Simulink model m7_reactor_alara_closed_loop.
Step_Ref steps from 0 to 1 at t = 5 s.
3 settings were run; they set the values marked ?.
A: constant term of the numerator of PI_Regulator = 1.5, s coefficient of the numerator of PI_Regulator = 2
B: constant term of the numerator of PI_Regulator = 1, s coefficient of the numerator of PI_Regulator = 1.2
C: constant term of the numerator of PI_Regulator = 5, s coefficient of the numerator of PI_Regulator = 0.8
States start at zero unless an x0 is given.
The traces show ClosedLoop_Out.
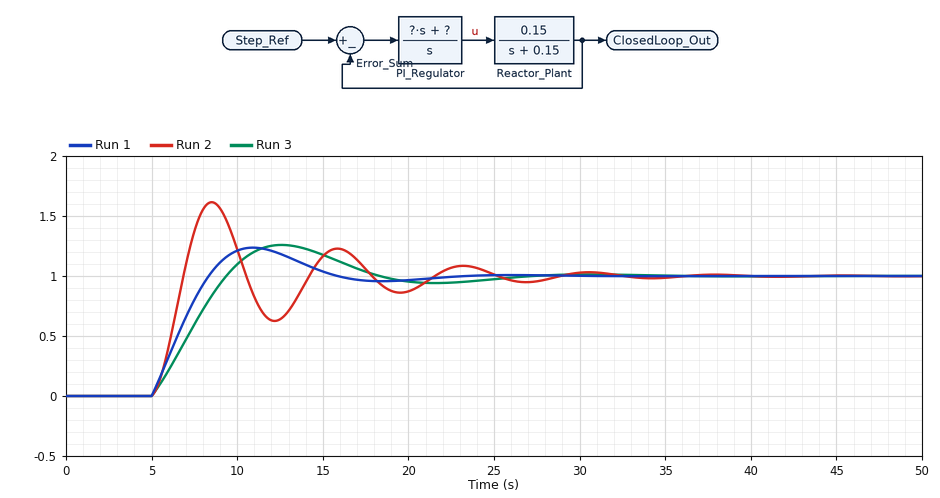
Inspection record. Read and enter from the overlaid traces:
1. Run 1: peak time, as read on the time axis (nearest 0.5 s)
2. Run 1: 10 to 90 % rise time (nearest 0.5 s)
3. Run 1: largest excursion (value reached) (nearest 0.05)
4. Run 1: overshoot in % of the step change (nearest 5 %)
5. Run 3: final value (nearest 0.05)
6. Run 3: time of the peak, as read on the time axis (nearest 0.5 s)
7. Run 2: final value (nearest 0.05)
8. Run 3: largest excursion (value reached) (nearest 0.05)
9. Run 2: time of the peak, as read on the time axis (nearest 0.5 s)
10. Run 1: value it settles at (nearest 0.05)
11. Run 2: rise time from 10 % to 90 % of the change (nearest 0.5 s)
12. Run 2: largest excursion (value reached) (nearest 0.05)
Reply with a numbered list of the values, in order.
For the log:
1. 11.0 s
2. 2.5 s
3. 1.25
4. 25 %
5. 1.00
6. 12.5 s
7. 1.00
8. 1.25
9. 8.5 s
10. 1.00
11. 1.5 s
12. 1.60
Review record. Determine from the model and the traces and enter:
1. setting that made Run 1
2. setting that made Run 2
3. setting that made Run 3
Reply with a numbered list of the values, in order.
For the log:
1. A
2. C
3. B
